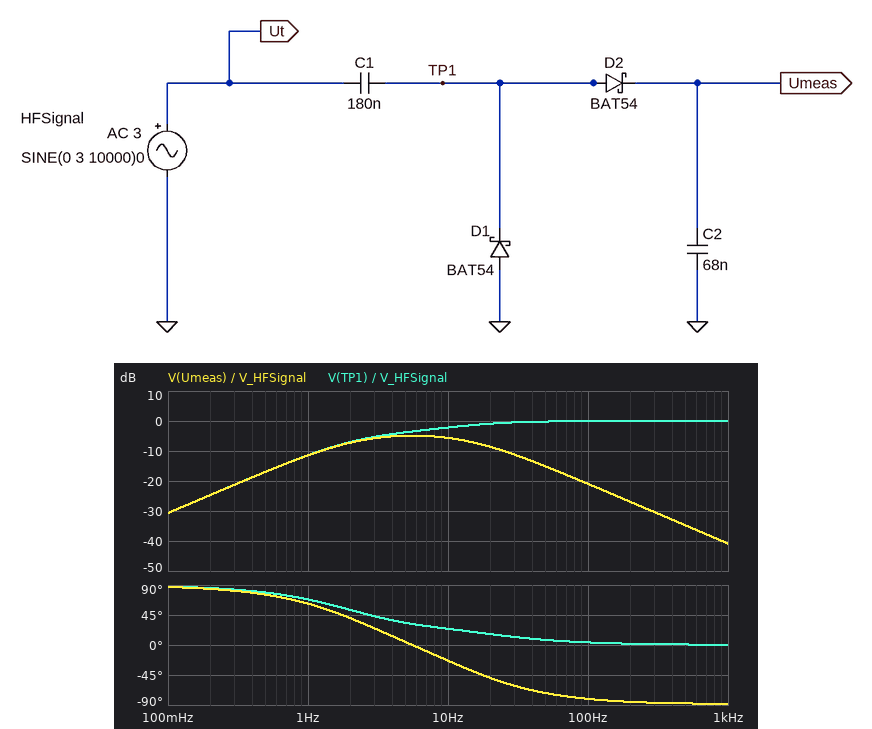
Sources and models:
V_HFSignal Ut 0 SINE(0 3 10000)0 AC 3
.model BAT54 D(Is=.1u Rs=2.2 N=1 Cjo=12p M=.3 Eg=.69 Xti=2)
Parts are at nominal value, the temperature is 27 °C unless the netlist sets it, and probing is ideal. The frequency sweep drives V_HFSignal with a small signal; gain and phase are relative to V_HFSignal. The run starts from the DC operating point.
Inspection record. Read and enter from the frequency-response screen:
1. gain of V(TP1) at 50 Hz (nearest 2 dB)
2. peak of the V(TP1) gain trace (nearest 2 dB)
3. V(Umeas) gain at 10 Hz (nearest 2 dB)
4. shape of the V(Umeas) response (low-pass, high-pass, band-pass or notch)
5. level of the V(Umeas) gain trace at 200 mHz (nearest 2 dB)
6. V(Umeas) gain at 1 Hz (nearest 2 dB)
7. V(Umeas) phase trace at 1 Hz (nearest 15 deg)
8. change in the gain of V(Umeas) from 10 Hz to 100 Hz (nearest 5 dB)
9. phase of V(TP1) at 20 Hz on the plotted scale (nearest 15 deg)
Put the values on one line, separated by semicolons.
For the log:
0 dB; 0 dB; -6 dB; band-pass; -24 dB; -12 dB; 60 deg; -15 dB; 15 deg
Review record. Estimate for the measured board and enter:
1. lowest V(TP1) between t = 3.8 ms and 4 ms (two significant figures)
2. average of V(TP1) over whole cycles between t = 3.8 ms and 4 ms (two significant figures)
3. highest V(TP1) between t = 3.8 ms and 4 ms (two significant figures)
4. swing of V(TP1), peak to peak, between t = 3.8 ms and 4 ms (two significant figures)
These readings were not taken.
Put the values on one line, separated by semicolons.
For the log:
-170 mV; 2.8 V; 5.8 V; 6.0 V
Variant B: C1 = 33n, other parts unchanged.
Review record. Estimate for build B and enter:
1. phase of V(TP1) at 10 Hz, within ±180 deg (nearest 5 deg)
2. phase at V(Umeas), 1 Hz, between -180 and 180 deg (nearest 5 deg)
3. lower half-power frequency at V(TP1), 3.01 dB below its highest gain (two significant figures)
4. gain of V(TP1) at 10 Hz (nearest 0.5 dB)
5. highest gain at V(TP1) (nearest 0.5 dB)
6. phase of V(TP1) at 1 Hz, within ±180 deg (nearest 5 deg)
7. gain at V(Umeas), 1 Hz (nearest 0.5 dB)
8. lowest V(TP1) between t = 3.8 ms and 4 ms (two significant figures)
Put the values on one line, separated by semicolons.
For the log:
55 deg; 75 deg; 41 Hz; -11.0 dB; 0 dB; 80 deg; -25.5 dB; -160 mV
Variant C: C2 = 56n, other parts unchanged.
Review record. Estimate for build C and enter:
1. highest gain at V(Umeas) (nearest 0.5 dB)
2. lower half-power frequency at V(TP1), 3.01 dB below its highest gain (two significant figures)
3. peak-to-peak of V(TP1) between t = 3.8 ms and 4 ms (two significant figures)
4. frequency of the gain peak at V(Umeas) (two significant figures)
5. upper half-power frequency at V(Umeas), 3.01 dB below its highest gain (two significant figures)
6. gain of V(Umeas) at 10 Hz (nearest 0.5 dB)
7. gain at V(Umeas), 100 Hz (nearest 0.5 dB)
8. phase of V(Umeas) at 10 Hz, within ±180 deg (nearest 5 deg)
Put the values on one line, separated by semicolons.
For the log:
-4.0 dB; 6.2 Hz; 6.0 V; 6.1 Hz; 20 Hz; -4.5 dB; -19.5 dB; -20 deg
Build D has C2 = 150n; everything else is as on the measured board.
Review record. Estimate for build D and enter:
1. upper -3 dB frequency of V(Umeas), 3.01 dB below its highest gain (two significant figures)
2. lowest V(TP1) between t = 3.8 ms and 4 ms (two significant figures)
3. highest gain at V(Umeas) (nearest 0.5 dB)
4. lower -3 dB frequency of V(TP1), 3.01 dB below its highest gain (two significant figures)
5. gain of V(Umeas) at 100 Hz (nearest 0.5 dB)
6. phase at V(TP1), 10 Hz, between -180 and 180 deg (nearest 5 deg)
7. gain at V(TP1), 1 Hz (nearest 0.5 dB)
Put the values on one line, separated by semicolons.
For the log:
12 Hz; -180 mV; -8.5 dB; 7.8 Hz; -28.0 dB; 30 deg; -12.0 dB
